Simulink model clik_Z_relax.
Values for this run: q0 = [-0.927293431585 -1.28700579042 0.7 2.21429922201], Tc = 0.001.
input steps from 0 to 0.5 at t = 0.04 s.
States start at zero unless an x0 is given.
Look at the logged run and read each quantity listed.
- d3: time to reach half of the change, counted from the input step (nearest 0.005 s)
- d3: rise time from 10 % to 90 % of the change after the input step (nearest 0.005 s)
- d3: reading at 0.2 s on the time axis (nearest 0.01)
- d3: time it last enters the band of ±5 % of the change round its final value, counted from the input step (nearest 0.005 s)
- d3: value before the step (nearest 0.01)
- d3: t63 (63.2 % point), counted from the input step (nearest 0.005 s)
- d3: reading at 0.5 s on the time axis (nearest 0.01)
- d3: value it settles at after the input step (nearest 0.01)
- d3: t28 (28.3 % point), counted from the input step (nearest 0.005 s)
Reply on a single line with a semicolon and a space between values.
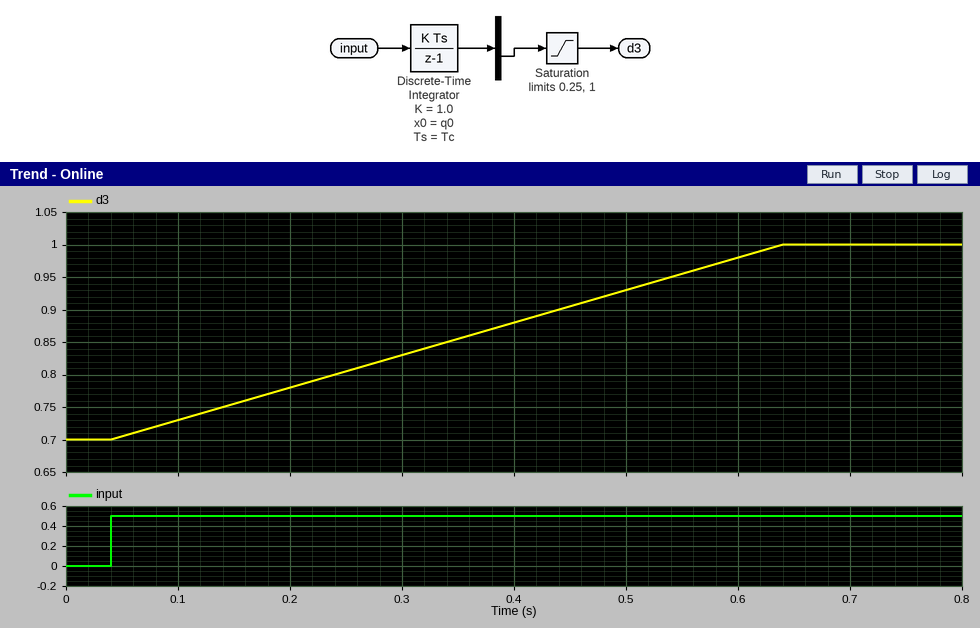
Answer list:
0.300 s; 0.480 s; 0.78; 0.570 s; 0.70; 0.380 s; 0.93; 1.00; 0.170 s
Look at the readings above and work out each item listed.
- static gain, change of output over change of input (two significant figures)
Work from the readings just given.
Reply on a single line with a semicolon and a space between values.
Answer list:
0.60
